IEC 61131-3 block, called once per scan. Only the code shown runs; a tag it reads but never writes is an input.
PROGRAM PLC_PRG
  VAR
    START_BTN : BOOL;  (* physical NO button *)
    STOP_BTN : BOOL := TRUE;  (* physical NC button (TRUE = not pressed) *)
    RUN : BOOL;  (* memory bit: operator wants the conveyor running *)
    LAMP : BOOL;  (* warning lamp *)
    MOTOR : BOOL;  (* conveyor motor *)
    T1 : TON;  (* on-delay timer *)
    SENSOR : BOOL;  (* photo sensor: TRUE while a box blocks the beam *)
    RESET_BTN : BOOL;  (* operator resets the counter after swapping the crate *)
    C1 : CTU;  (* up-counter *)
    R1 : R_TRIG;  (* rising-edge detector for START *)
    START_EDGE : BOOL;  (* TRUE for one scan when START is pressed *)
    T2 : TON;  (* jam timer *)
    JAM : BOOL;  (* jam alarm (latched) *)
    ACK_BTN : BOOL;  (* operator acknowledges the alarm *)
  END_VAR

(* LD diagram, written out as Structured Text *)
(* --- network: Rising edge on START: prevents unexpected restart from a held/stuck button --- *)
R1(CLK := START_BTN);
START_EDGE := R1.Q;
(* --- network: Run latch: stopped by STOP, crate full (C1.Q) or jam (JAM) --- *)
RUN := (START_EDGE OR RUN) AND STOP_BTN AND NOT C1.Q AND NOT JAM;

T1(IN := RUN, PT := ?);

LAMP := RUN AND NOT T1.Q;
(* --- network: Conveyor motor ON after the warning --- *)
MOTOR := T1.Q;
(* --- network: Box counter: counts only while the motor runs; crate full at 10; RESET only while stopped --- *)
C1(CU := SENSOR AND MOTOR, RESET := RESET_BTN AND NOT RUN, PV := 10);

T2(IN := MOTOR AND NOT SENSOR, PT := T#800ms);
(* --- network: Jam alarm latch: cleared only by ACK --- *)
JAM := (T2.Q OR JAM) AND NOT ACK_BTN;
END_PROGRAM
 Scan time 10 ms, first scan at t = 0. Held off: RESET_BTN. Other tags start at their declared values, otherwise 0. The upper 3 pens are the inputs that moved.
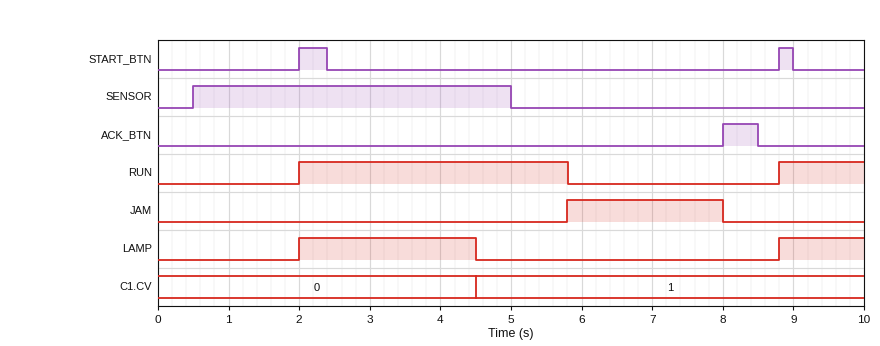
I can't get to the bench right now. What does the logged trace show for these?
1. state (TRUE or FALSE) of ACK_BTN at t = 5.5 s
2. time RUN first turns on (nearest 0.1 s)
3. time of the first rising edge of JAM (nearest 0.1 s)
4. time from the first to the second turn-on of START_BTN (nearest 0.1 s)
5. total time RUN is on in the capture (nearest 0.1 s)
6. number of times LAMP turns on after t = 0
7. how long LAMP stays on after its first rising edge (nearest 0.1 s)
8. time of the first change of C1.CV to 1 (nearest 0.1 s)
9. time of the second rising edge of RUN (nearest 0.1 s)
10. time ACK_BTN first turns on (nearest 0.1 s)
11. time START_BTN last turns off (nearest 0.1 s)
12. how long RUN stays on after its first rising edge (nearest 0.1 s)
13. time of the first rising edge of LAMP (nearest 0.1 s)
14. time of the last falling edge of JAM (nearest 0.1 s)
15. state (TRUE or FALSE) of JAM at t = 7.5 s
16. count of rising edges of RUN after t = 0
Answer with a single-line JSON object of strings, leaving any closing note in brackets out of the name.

{"state (TRUE or FALSE) of ACK_BTN at t = 5.5 s": "FALSE", "time RUN first turns on": "2.0 s", "time of the first rising edge of JAM": "5.8 s", "time from the first to the second turn-on of START_BTN": "6.8 s", "total time RUN is on in the capture": "5.0 s", "number of times LAMP turns on after t = 0": "2", "how long LAMP stays on after its first rising edge": "2.5 s", "time of the first change of C1.CV to 1": "4.5 s", "time of the second rising edge of RUN": "8.8 s", "time ACK_BTN first turns on": "8.0 s", "time START_BTN last turns off": "9.0 s", "how long RUN stays on after its first rising edge": "3.8 s", "time of the first rising edge of LAMP": "2.0 s", "time of the last falling edge of JAM": "8.0 s", "state (TRUE or FALSE) of JAM at t = 7.5 s": "TRUE", "count of rising edges of RUN after t = 0": "2"}
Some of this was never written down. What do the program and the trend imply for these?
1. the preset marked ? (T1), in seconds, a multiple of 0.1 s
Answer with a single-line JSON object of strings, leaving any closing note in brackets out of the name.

{"the preset marked ? (T1), in seconds, a multiple of 0.1 s": "2.5 s"}
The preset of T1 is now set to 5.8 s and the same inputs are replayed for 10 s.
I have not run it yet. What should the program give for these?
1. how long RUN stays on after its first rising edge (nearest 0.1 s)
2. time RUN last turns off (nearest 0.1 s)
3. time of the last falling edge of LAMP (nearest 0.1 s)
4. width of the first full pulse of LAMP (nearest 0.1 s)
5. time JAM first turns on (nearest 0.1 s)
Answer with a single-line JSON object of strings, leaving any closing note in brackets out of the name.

{"how long RUN stays on after its first rising edge": "6.6 s", "time RUN last turns off": "8.6 s", "time of the last falling edge of LAMP": "7.8 s", "width of the first full pulse of LAMP": "5.8 s", "time JAM first turns on": "8.6 s"}
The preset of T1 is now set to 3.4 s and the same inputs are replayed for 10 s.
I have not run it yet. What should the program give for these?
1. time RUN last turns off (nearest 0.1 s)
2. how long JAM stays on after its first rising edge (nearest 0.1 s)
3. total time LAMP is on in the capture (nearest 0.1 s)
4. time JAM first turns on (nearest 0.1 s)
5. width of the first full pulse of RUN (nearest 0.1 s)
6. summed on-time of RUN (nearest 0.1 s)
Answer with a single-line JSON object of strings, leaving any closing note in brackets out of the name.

{"time RUN last turns off": "6.2 s", "how long JAM stays on after its first rising edge": "1.8 s", "total time LAMP is on in the capture": "4.6 s", "time JAM first turns on": "6.2 s", "width of the first full pulse of RUN": "4.2 s", "summed on-time of RUN": "5.4 s"}
